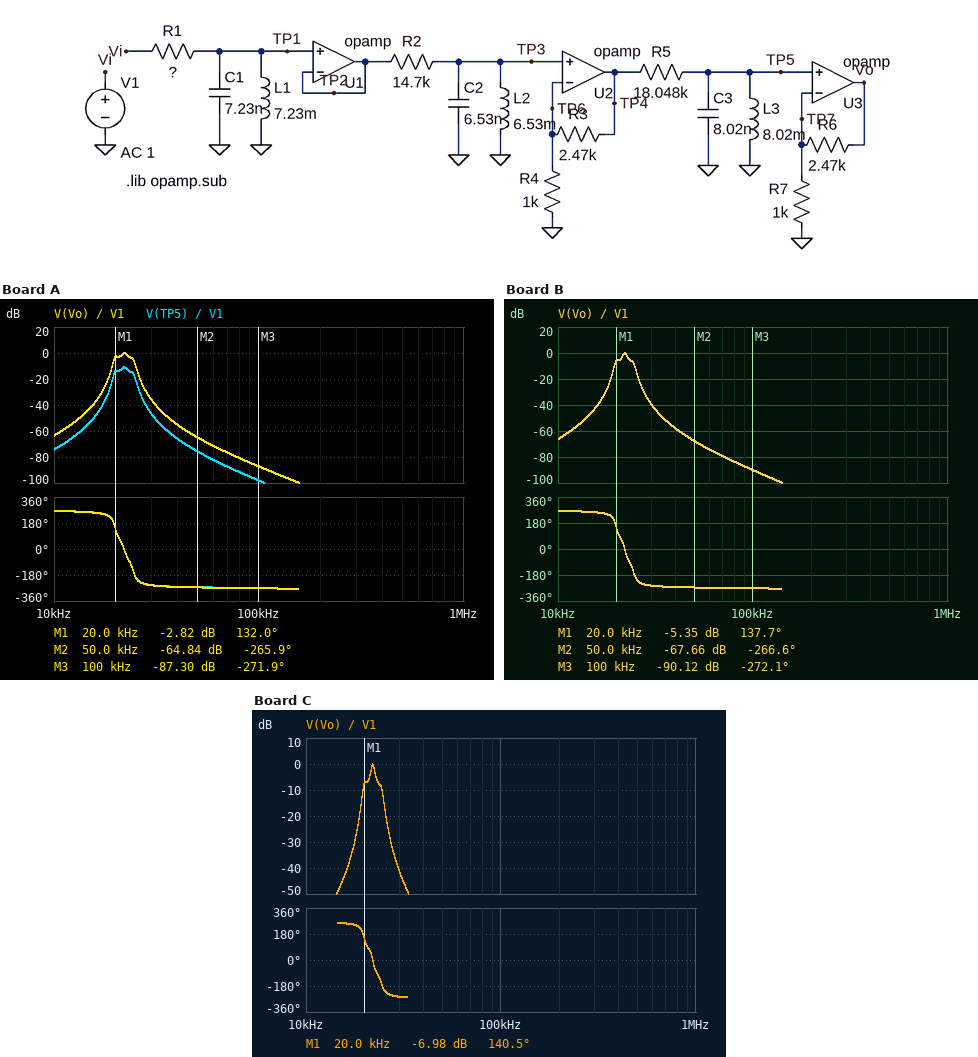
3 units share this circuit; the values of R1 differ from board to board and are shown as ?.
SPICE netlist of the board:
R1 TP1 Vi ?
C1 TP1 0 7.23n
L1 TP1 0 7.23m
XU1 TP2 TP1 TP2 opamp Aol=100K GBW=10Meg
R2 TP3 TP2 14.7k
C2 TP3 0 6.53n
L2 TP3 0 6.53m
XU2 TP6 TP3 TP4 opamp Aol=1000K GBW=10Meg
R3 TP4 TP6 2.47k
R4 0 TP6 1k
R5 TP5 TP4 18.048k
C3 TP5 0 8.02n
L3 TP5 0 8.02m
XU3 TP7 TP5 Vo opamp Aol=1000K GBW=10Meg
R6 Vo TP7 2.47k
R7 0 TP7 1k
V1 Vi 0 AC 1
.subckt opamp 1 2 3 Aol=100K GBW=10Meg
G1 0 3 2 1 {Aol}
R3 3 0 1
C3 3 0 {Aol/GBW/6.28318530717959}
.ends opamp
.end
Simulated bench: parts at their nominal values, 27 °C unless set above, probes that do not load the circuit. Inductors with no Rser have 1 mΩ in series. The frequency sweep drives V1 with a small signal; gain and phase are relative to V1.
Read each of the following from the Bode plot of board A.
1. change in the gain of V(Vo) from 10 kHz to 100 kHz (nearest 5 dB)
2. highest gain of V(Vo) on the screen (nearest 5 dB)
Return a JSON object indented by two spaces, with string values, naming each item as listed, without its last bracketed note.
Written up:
{
  "change in the gain of V(Vo) from 10 kHz to 100 kHz": "-25 dB",
  "highest gain of V(Vo) on the screen": "0 dB"
}
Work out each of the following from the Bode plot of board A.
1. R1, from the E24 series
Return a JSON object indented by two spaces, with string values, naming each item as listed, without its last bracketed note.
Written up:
{
  "R1, from the E24 series": "13 kΩ"
}
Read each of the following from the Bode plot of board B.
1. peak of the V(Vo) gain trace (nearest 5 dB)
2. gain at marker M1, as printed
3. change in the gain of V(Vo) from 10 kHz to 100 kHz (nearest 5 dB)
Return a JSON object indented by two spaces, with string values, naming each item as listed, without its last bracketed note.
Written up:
{
  "peak of the V(Vo) gain trace": "0 dB",
  "gain at marker M1, as printed": "-5.35 dB",
  "change in the gain of V(Vo) from 10 kHz to 100 kHz": "-25 dB"
}
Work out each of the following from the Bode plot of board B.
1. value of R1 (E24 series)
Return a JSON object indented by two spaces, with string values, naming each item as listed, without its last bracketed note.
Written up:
{
  "value of R1": "18 kΩ"
}
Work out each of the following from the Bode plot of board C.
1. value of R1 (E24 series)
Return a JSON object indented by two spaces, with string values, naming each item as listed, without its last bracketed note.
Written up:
{
  "value of R1": "22 kΩ"
}
